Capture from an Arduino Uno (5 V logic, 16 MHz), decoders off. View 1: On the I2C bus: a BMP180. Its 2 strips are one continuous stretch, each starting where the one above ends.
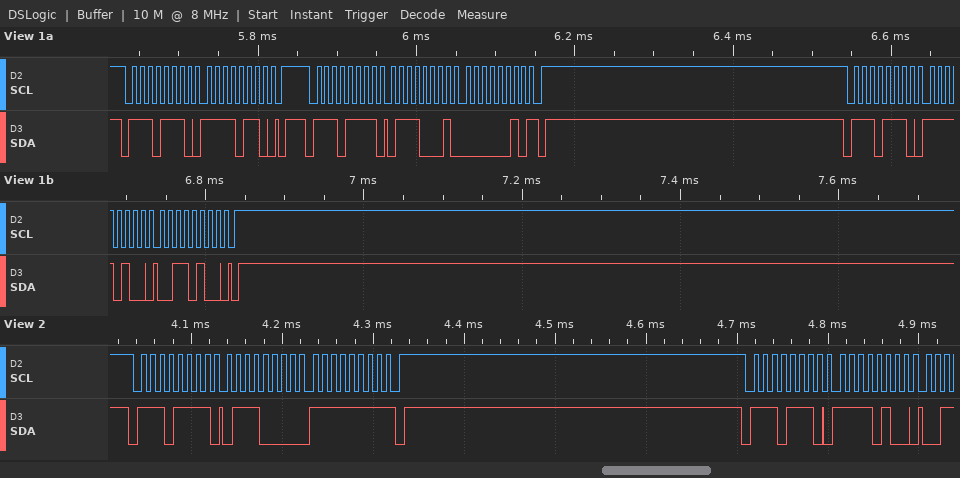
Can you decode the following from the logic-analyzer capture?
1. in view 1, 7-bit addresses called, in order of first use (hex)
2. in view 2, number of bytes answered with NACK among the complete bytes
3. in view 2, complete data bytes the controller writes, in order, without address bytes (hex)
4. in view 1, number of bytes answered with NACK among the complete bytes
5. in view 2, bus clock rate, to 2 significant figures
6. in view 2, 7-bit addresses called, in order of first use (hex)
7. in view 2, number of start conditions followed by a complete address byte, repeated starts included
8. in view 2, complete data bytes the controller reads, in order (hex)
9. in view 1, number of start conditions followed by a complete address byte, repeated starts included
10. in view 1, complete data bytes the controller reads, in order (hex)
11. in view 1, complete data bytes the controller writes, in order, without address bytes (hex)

0x77
1
F4
1
100 kHz
0x77
2
70 FF
3
71 02
F6 F4 34
